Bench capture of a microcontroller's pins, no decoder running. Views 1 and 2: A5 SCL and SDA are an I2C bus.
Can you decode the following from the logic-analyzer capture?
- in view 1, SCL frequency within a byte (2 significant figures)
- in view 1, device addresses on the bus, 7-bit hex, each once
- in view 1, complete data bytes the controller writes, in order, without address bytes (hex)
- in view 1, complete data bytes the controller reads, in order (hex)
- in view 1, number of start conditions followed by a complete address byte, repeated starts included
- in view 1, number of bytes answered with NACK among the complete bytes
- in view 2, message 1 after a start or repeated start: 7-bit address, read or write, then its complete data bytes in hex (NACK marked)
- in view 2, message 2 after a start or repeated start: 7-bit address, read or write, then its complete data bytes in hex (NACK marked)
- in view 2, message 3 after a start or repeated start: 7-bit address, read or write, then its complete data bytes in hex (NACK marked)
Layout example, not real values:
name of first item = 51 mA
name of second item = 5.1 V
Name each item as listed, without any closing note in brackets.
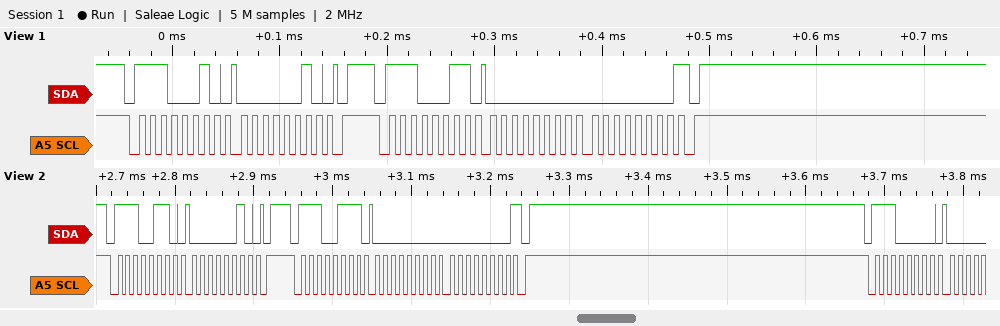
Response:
in view 1, SCL frequency within a byte = 100 kHz
in view 1, device addresses on the bus, 7-bit hex, each once = 0x71
in view 1, complete data bytes the controller writes, in order, without address bytes = 02
in view 1, complete data bytes the controller reads, in order = 00 00
in view 1, number of start conditions followed by a complete address byte, repeated starts included = 2
in view 1, number of bytes answered with NACK among the complete bytes = 1
in view 2, message 1 after a start or repeated start: 7-bit address, read or write, then its complete data bytes in hex = 0x73 write: 02
in view 2, message 2 after a start or repeated start: 7-bit address, read or write, then its complete data bytes in hex = 0x73 read: 00 00 NACK
in view 2, message 3 after a start or repeated start: 7-bit address, read or write, then its complete data bytes in hex = 0x70 write
